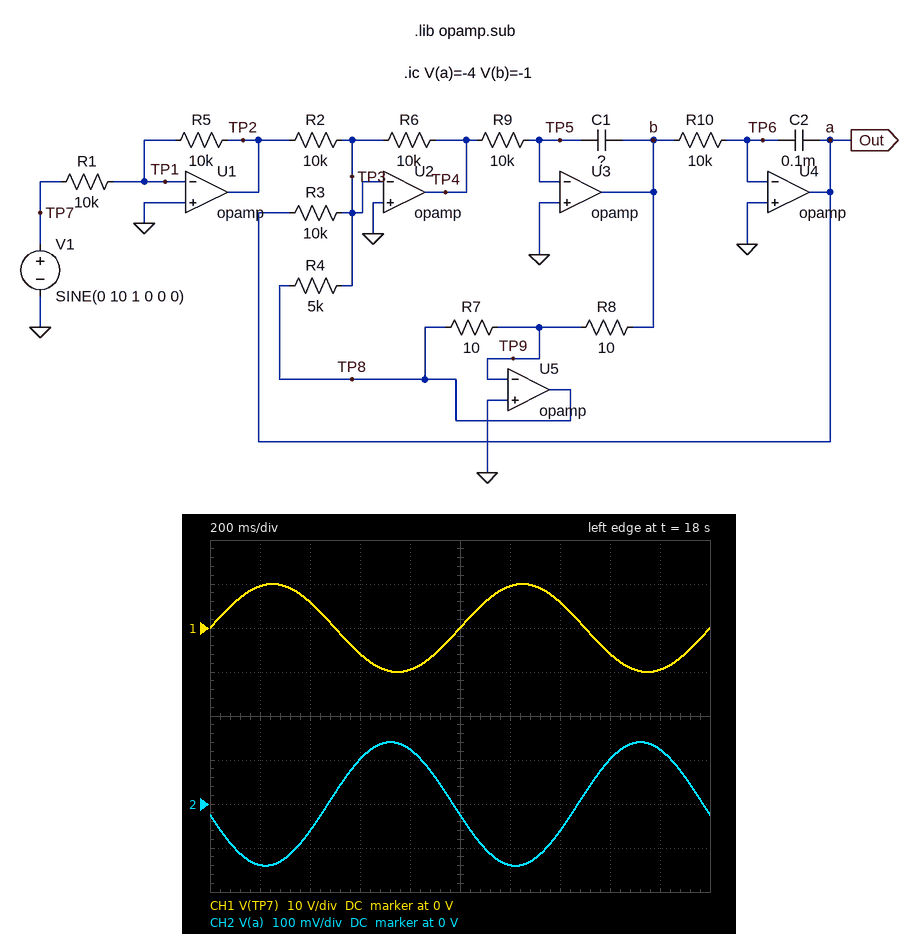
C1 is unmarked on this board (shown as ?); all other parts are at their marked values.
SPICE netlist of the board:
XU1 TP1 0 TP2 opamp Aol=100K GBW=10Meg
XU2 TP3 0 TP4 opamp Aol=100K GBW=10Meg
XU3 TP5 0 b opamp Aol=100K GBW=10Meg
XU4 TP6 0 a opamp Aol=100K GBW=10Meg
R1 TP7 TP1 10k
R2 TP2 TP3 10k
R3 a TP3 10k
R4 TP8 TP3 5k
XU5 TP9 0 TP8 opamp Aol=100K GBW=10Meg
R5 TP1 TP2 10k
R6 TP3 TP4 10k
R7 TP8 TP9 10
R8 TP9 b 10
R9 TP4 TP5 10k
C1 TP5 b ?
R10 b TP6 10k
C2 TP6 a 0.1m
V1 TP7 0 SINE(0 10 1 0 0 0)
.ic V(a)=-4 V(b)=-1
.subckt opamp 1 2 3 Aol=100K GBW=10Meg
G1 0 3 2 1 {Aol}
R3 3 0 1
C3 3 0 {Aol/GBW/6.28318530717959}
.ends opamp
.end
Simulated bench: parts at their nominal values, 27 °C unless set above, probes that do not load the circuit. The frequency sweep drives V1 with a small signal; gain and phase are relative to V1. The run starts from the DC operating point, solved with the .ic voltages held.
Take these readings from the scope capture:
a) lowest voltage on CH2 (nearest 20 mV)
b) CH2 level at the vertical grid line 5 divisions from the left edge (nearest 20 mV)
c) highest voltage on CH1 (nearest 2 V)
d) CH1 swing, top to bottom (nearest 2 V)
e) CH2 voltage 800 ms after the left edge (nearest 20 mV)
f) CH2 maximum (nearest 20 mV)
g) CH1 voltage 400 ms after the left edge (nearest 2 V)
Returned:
-140 mV
-20 mV
10 V
20 V
120 mV
140 mV
6 V
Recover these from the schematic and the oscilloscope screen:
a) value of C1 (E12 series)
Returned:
180 µF
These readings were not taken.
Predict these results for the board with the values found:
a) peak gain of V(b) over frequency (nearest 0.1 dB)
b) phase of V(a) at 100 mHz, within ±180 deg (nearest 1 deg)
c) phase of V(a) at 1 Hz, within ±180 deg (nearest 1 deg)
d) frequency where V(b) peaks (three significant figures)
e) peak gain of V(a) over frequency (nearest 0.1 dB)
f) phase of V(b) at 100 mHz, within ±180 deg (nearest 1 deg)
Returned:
-6.0 dB
-77 deg
-170 deg
119 mHz
0 dB
-167 deg
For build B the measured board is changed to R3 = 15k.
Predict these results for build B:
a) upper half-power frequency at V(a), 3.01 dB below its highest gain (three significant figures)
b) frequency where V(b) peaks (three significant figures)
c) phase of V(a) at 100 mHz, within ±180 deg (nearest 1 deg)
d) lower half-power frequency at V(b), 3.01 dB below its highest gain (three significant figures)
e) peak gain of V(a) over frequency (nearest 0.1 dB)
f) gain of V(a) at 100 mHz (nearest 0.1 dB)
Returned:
70.9 mHz
96.9 mHz
-92 deg
42.7 mHz
3.5 dB
-2.0 dB
